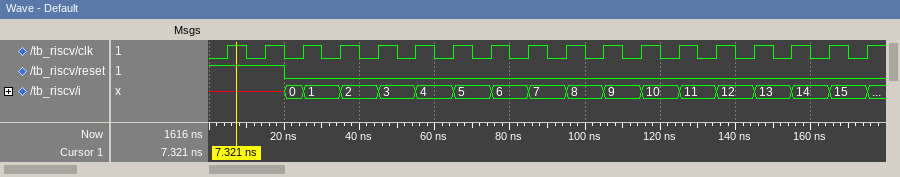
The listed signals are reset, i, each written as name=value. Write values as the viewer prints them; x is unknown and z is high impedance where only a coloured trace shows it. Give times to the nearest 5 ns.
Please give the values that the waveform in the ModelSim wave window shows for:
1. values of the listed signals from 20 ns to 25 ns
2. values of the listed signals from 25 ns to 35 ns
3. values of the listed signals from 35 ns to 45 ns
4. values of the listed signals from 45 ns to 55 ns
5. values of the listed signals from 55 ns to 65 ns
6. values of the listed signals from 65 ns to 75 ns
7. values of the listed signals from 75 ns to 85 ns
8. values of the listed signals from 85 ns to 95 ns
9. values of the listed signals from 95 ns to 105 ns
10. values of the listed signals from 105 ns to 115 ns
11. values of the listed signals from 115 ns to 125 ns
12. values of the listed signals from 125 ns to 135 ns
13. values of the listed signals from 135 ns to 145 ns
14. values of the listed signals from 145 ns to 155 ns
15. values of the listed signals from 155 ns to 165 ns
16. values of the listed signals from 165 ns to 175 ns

reset=0, i=0
reset=0, i=1
reset=0, i=2
reset=0, i=3
reset=0, i=4
reset=0, i=5
reset=0, i=6
reset=0, i=7
reset=0, i=8
reset=0, i=9
reset=0, i=10
reset=0, i=11
reset=0, i=12
reset=0, i=13
reset=0, i=14
reset=0, i=15
